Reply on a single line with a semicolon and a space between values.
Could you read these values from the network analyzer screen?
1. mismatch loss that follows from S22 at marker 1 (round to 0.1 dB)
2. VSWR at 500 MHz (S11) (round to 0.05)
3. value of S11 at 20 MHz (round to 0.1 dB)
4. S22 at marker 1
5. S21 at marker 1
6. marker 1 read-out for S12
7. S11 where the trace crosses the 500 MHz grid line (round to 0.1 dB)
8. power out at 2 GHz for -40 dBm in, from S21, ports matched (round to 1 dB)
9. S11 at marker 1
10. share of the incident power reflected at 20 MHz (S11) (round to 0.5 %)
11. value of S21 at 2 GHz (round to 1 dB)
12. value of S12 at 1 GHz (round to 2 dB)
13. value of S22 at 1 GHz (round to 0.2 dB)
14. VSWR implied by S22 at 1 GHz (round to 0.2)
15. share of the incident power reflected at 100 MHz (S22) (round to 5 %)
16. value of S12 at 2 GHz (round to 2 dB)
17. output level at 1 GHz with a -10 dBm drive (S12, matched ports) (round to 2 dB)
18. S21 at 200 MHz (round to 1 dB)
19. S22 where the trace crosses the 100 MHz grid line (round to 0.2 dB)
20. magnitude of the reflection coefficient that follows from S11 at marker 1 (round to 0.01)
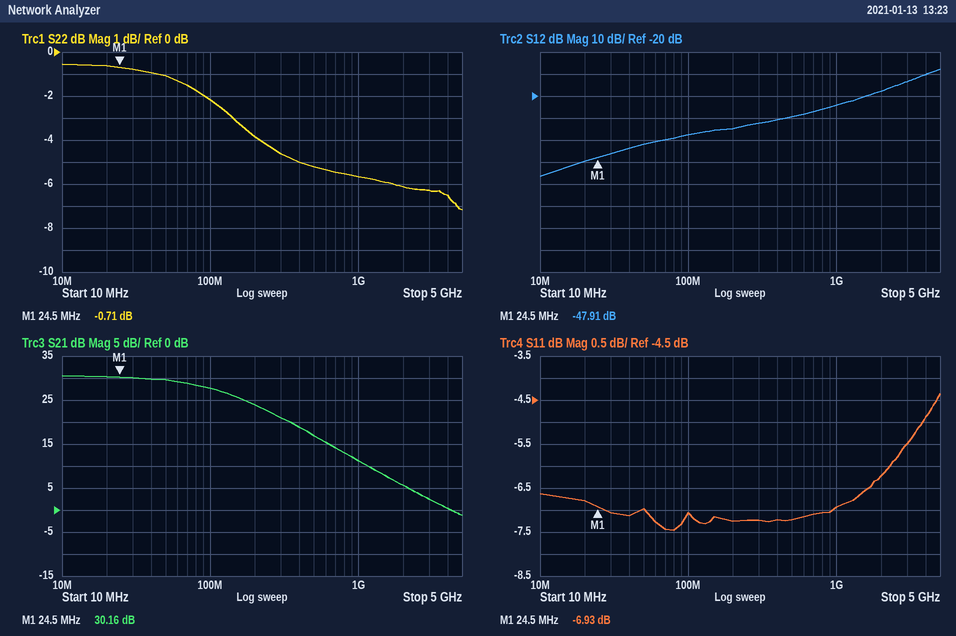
8.2 dB; 2.55; -6.8 dB; -0.71 dB; 30.16 dB; -47.91 dB; -7.2 dB; -34 dBm; -6.93 dB; 21.0 %; 6 dB; -24 dB; -5.6 dB; 3.2; 60 %; -18 dB; -34 dBm; 24 dB; -2.2 dB; 0.45
